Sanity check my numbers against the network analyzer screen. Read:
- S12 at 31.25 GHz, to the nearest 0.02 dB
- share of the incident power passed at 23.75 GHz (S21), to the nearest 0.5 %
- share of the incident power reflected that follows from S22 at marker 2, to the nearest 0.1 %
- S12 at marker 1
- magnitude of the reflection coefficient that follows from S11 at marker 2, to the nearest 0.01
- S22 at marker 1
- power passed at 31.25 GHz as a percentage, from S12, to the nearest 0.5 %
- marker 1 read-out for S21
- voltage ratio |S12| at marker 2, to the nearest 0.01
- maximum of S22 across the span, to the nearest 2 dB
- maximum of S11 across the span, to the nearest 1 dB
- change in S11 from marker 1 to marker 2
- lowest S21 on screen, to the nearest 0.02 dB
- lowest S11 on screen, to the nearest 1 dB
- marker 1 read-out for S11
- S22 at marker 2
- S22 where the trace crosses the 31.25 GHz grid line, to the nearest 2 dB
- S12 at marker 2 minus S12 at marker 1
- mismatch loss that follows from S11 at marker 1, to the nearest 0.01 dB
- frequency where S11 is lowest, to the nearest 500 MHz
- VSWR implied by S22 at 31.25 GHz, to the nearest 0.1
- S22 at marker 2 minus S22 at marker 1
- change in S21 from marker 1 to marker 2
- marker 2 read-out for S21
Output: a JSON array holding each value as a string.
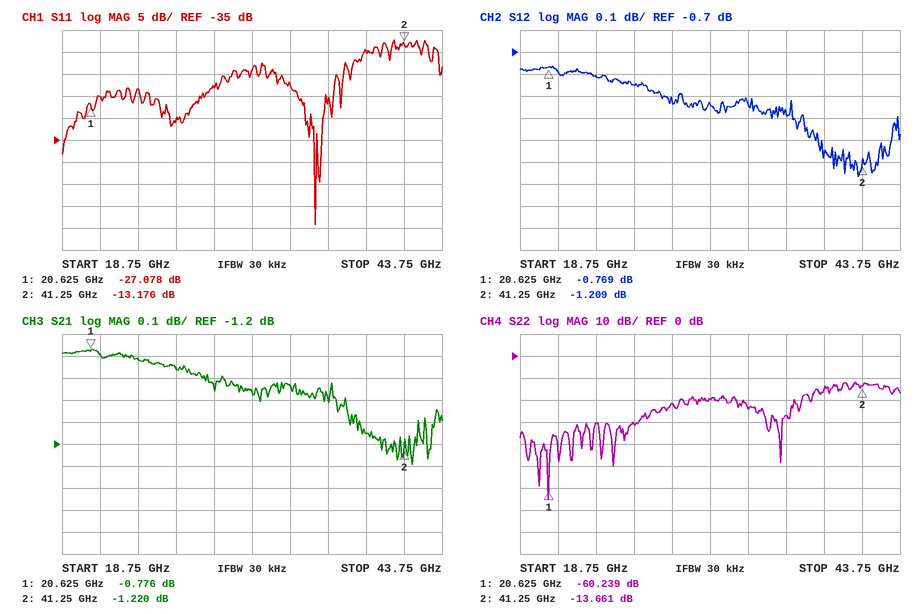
["-0.94 dB", "83.0 %", "4.3 %", "-0.769 dB", "0.22", "-60.239 dB", "80.5 %", "-0.776 dB", "0.87", "-12 dB", "-12 dB", "13.902 dB", "-1.30 dB", "-54 dB", "-27.078 dB", "-13.661 dB", "-20 dB", "-0.440 dB", "0.01 dB", "35.5 GHz", "1.2", "46.578 dB", "-0.444 dB", "-1.220 dB"]
